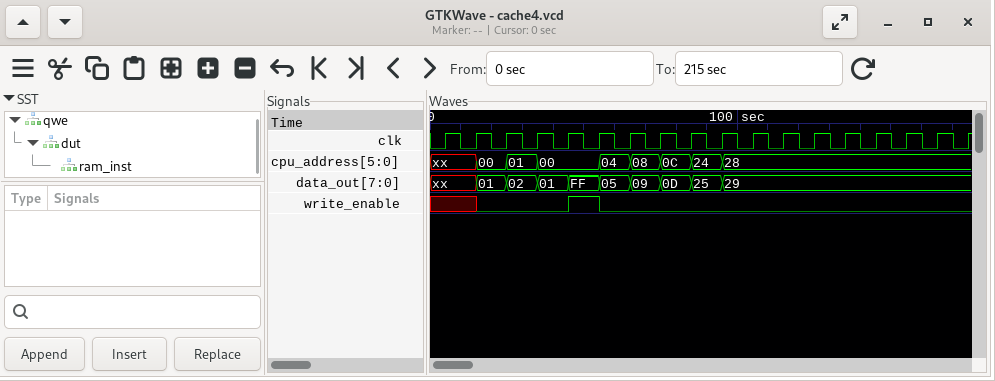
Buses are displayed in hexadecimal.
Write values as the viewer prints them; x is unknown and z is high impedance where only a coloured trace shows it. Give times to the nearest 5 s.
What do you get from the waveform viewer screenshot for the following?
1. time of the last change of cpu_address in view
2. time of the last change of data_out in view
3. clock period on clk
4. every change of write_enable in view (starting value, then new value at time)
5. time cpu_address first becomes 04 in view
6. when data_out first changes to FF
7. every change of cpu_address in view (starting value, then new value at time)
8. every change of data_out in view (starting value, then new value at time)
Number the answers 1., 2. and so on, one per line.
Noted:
1. 95 s
2. 95 s
3. 10 s
4. x, 0 at 15 s, 1 at 45 s, 0 at 55 s
5. 55 s
6. 45 s
7. xx, 00 at 15 s, 01 at 25 s, 00 at 35 s, 04 at 55 s, 08 at 65 s, 0C at 75 s, 24 at 85 s, 28 at 95 s
8. xx, 01 at 15 s, 02 at 25 s, 01 at 35 s, FF at 45 s, 05 at 55 s, 09 at 65 s, 0D at 75 s, 25 at 85 s, 29 at 95 s
